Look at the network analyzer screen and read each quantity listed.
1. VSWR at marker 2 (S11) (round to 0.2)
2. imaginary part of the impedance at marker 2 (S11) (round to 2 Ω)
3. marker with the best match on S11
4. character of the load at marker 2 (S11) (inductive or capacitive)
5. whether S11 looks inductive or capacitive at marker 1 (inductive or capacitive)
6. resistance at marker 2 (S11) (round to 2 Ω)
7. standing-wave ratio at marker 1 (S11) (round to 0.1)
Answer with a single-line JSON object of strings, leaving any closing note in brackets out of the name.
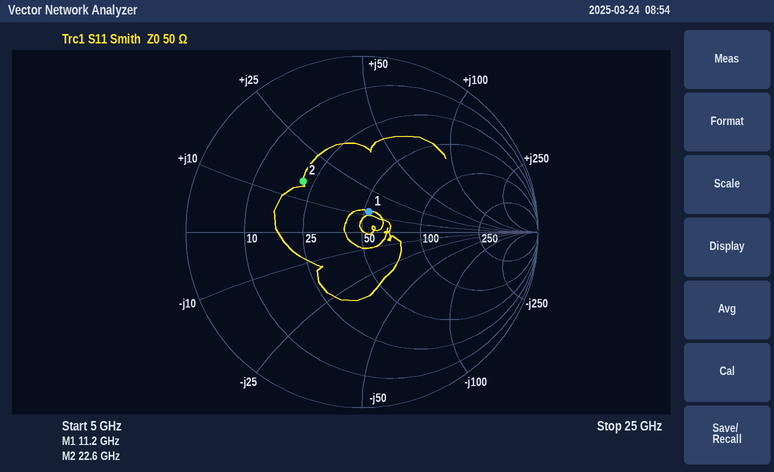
{"VSWR at marker 2 (S11)": "2.6", "imaginary part of the impedance at marker 2 (S11)": "+16 Ω", "marker with the best match on S11": "marker 1", "character of the load at marker 2 (S11)": "inductive", "whether S11 looks inductive or capacitive at marker 1": "inductive", "resistance at marker 2 (S11)": "22 Ω", "standing-wave ratio at marker 1 (S11)": "1.3"}
